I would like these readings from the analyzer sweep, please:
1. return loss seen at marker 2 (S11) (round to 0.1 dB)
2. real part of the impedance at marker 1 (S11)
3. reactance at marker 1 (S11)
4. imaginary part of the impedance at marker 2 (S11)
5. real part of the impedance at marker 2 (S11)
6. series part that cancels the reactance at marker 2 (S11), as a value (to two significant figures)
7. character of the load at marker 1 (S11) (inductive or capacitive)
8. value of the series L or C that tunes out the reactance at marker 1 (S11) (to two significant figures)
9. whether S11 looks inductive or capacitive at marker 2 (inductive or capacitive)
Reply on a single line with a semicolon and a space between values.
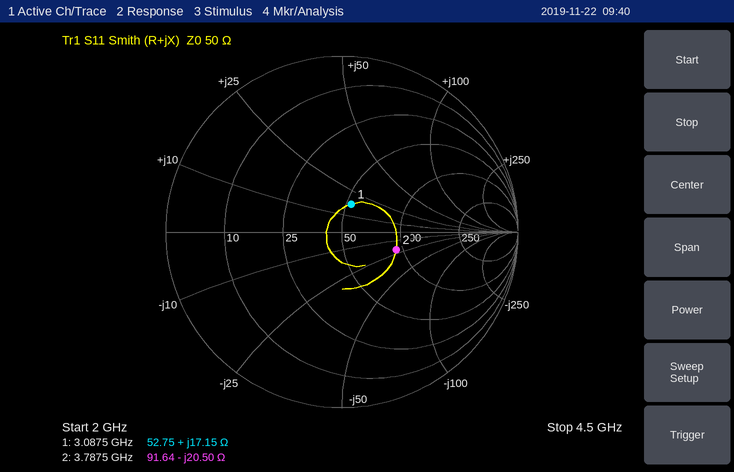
9.8 dB; 52.75 Ω; +17.15 Ω; -20.50 Ω; 91.64 Ω; 860 pH; inductive; 3.0 pF; capacitive
